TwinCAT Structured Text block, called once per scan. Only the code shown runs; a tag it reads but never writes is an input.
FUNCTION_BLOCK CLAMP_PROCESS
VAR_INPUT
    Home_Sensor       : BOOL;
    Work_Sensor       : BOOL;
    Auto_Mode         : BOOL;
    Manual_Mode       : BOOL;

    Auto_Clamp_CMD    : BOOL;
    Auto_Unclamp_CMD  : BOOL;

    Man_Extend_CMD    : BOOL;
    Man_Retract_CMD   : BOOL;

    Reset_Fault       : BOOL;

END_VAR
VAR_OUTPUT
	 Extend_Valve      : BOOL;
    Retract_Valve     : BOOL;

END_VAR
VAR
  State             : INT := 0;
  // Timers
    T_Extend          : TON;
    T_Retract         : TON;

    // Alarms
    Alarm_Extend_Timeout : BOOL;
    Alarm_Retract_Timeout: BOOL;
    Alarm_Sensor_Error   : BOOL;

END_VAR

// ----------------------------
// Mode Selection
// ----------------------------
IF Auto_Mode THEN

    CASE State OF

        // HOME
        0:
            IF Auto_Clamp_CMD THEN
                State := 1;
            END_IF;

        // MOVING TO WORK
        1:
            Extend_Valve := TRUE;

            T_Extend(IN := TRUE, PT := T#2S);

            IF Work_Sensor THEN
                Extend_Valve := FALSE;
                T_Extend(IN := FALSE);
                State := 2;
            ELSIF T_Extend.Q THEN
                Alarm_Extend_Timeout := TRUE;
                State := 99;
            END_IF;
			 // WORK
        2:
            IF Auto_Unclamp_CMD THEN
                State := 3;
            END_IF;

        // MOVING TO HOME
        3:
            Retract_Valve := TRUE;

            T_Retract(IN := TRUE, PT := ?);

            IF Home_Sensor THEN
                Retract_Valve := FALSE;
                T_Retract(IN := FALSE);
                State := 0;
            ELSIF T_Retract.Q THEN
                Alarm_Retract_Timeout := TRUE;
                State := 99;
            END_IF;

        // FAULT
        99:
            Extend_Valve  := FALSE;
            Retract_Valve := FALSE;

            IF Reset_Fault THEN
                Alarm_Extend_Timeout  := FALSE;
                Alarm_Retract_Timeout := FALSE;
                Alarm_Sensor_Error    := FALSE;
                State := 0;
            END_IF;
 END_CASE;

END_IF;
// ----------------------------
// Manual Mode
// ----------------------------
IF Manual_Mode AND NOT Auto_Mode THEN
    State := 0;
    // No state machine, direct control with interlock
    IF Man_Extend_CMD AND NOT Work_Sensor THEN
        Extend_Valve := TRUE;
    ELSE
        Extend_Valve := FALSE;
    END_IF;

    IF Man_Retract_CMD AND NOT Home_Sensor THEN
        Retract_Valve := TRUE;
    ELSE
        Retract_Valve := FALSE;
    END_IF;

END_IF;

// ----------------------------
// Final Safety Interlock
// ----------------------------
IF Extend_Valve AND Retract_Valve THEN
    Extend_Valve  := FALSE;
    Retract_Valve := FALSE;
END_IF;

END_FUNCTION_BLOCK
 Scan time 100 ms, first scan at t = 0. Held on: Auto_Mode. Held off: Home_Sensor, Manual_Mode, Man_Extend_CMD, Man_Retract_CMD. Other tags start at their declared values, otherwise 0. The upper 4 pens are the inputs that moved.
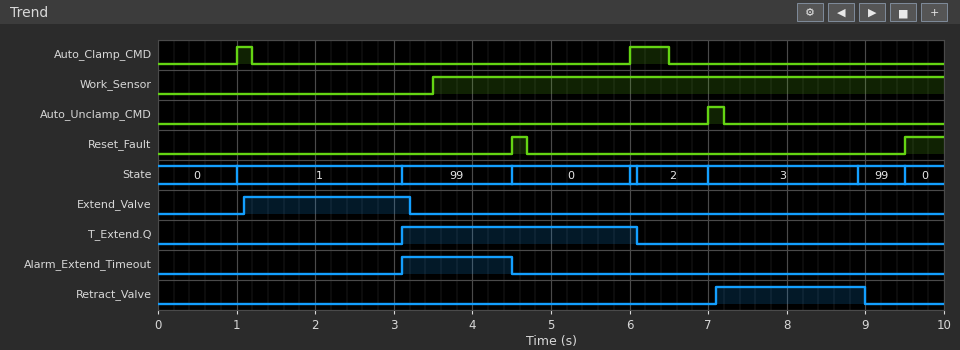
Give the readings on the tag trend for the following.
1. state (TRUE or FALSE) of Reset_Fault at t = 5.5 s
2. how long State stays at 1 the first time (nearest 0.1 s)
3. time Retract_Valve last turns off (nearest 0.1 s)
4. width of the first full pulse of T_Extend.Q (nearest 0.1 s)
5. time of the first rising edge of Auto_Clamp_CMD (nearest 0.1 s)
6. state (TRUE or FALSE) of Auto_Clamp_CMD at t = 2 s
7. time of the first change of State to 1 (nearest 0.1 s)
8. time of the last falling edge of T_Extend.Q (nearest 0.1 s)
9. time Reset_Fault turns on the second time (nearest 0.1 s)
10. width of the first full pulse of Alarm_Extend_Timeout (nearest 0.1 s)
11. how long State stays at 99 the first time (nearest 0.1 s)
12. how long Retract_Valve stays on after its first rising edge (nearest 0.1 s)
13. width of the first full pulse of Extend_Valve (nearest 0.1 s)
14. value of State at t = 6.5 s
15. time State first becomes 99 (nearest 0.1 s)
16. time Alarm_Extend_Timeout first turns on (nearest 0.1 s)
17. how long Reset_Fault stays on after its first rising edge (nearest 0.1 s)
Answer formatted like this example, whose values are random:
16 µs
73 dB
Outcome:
FALSE
2.1 s
9.0 s
3.0 s
1.0 s
FALSE
1.0 s
6.1 s
9.5 s
1.4 s
1.4 s
1.9 s
2.1 s
2
3.1 s
3.1 s
0.2 s
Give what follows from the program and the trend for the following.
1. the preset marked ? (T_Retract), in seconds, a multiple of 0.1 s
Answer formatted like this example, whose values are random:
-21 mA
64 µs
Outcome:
1.8 s
